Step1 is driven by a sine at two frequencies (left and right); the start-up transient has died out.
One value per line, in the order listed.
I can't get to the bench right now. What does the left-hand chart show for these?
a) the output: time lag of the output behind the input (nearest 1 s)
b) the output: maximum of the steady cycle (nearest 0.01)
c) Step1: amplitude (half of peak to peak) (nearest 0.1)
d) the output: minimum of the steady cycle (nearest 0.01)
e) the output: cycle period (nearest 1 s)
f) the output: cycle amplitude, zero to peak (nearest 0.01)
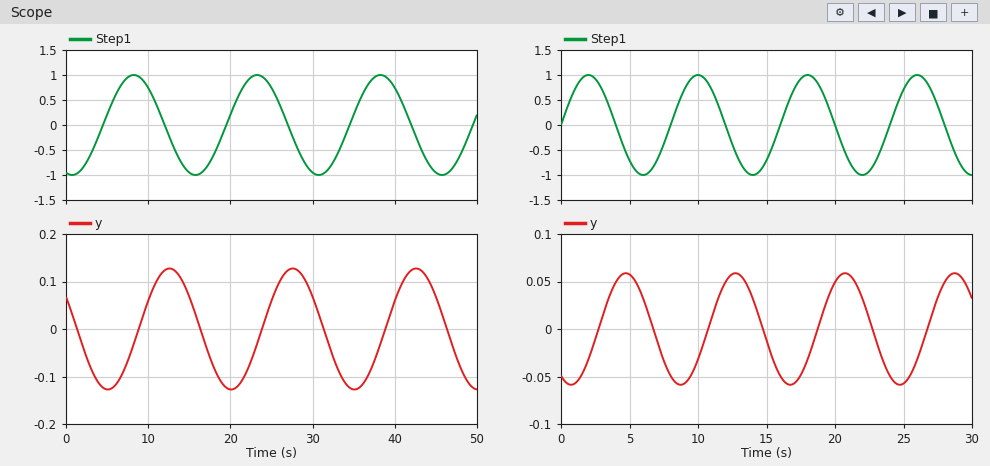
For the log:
4 s
0.13
1.0
-0.13
15 s
0.13
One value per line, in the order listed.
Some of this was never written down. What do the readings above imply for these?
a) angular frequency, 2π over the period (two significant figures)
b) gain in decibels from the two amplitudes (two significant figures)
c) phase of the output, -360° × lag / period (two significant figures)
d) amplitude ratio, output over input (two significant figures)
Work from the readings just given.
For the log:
0.42 rad/s
-18 dB
-96°
0.13
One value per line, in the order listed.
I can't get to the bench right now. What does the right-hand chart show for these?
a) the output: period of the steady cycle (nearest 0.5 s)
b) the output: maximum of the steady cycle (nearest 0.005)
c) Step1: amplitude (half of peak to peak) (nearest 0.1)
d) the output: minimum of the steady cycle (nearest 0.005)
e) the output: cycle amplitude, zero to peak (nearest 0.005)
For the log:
8.0 s
0.060
1.0
-0.060
0.060
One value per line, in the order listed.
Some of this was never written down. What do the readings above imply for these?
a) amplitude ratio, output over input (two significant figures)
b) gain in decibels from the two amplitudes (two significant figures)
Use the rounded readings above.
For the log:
0.060
-24 dB
